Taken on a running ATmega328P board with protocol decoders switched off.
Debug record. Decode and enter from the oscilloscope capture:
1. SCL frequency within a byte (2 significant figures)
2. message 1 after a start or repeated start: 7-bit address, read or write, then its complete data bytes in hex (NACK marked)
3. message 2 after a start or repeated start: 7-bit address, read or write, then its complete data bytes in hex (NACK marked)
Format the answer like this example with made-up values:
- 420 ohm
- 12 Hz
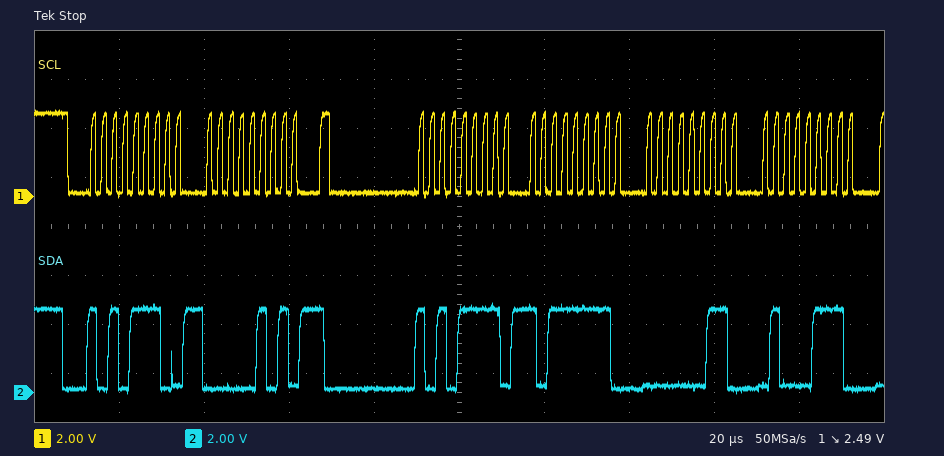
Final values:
- 400 kHz
- 0x57 write: 05
- 0x57 read: BF 03 47
